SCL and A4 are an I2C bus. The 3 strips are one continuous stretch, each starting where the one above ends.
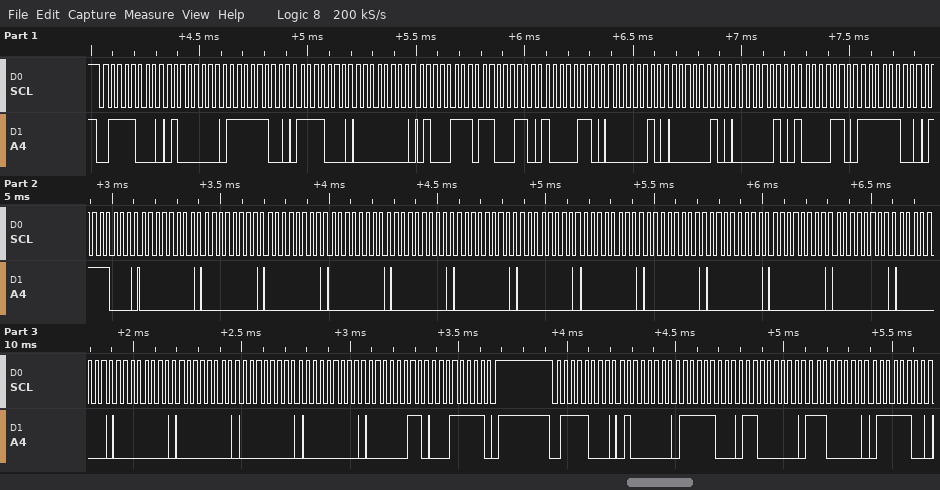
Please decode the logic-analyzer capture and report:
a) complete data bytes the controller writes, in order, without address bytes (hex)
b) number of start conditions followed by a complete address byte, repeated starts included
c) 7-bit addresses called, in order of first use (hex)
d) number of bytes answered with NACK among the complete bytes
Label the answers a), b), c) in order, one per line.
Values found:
a) 40 FC 78 00 47 C6 86 02 02 02 86 FC 78 00 00 00 00 00 00 00 00 00 00 00 00 00 00 00 00 00 03 1F 40 F8 C0 E0 7C
b) 2
c) 0x3C
d) 0
